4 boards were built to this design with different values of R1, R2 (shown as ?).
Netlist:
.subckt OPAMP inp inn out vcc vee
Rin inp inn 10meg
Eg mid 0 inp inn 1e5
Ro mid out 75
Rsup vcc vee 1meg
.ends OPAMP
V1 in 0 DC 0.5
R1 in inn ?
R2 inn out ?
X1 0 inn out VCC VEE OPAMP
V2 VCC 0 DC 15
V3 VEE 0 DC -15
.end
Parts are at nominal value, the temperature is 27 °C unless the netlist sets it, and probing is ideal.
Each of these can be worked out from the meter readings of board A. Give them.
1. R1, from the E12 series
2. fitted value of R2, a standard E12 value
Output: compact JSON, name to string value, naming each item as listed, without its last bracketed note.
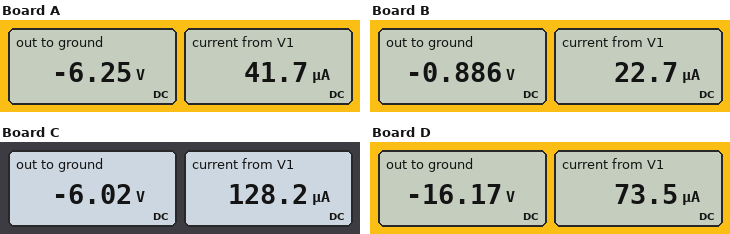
{"R1, from the E12 series": "12 kΩ", "fitted value of R2, a standard E12 value": "150 kΩ"}
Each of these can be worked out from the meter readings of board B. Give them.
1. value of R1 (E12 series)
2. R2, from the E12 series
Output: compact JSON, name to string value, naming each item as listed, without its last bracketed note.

{"value of R1": "22 kΩ", "R2, from the E12 series": "39 kΩ"}
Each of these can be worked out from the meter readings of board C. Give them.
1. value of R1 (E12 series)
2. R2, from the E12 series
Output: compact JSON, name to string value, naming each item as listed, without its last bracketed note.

{"value of R1": "3.9 kΩ", "R2, from the E12 series": "47 kΩ"}
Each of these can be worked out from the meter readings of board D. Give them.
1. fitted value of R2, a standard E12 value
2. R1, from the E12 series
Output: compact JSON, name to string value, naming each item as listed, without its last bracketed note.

{"fitted value of R2, a standard E12 value": "220 kΩ", "R1, from the E12 series": "6.8 kΩ"}
